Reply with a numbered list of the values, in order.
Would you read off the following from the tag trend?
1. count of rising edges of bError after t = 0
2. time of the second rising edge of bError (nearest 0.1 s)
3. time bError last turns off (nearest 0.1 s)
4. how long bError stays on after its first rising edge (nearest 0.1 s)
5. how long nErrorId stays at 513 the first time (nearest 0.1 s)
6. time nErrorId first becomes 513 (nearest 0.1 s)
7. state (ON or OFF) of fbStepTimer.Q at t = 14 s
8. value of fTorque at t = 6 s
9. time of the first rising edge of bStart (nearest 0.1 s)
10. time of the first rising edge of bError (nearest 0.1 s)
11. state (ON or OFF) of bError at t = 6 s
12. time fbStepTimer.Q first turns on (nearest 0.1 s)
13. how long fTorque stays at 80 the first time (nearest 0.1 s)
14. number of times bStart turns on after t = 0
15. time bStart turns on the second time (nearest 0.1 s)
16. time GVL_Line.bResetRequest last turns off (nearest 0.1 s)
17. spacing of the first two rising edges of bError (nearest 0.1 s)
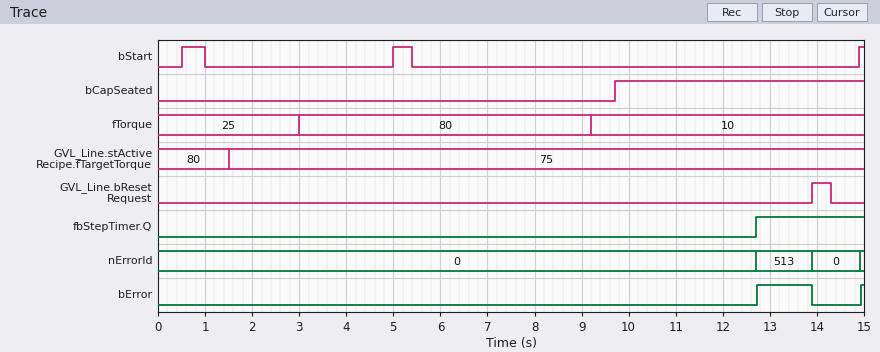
1. 2
2. 14.9 s
3. 13.9 s
4. 1.2 s
5. 1.2 s
6. 12.7 s
7. ON
8. 80
9. 0.5 s
10. 12.7 s
11. OFF
12. 12.7 s
13. 6.2 s
14. 3
15. 5.0 s
16. 14.3 s
17. 2.2 s
